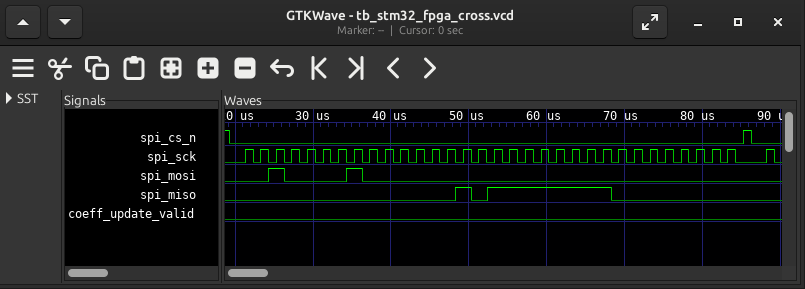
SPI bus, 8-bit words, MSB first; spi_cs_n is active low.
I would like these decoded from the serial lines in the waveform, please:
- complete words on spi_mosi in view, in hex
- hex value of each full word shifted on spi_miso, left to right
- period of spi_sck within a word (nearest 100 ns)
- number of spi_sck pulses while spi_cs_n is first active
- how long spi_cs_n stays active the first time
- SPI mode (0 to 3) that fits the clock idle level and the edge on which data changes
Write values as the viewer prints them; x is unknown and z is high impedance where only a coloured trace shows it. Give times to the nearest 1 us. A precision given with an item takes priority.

21, 00, 00, 00
00, 02, FF, 00
2000 ns
32
66 us
0
